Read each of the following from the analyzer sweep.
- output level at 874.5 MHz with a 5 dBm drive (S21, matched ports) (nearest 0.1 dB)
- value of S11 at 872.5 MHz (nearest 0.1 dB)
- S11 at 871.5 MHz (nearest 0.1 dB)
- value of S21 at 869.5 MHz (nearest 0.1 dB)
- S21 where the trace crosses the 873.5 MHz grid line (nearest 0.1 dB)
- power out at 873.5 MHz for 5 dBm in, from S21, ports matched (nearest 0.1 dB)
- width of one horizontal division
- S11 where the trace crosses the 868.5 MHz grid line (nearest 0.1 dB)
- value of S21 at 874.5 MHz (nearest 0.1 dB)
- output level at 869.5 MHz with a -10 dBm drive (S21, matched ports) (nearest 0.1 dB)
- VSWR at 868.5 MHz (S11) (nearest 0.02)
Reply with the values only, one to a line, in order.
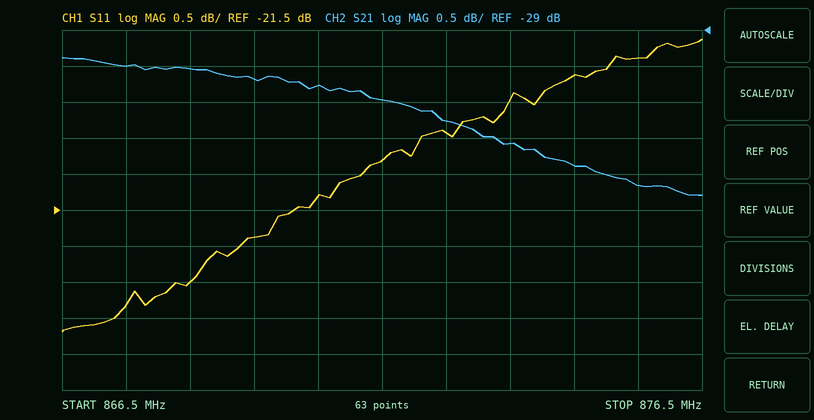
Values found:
-25.9 dBm
-20.4 dB
-20.8 dB
-29.7 dB
-30.6 dB
-25.6 dBm
1 MHz
-22.5 dB
-30.9 dB
-39.7 dBm
1.16
